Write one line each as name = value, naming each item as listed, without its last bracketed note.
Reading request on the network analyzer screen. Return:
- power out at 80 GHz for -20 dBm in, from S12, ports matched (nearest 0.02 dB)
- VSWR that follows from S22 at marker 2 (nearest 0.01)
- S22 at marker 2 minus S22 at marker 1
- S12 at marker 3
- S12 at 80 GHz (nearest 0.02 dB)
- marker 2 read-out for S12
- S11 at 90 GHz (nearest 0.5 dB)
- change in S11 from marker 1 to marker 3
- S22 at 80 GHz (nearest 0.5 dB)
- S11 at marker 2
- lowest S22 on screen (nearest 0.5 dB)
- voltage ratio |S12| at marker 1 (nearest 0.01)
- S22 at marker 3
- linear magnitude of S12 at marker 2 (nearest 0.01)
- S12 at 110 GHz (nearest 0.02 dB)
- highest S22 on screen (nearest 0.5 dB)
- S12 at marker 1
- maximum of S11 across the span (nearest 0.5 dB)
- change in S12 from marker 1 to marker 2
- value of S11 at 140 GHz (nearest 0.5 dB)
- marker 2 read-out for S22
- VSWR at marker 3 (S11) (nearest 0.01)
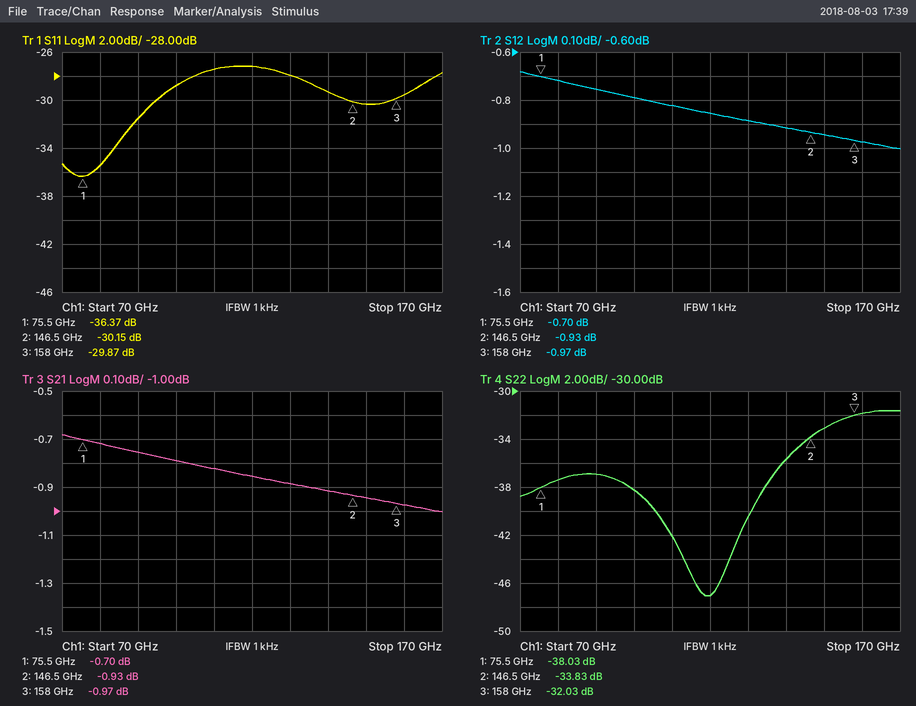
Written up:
power out at 80 GHz for -20 dBm in, from S12, ports matched = -20.72 dBm
VSWR that follows from S22 at marker 2 = 1.04
S22 at marker 2 minus S22 at marker 1 = 4.20 dB
S12 at marker 3 = -0.97 dB
S12 at 80 GHz = -0.72 dB
marker 2 read-out for S12 = -0.93 dB
S11 at 90 GHz = -31.5 dB
change in S11 from marker 1 to marker 3 = 6.50 dB
S22 at 80 GHz = -37.5 dB
S11 at marker 2 = -30.15 dB
lowest S22 on screen = -47.0 dB
voltage ratio |S12| at marker 1 = 0.92
S22 at marker 3 = -32.03 dB
linear magnitude of S12 at marker 2 = 0.90
S12 at 110 GHz = -0.82 dB
highest S22 on screen = -31.5 dB
S12 at marker 1 = -0.70 dB
maximum of S11 across the span = -27.0 dB
change in S12 from marker 1 to marker 2 = -0.23 dB
value of S11 at 140 GHz = -29.5 dB
marker 2 read-out for S22 = -33.83 dB
VSWR at marker 3 (S11) = 1.07
